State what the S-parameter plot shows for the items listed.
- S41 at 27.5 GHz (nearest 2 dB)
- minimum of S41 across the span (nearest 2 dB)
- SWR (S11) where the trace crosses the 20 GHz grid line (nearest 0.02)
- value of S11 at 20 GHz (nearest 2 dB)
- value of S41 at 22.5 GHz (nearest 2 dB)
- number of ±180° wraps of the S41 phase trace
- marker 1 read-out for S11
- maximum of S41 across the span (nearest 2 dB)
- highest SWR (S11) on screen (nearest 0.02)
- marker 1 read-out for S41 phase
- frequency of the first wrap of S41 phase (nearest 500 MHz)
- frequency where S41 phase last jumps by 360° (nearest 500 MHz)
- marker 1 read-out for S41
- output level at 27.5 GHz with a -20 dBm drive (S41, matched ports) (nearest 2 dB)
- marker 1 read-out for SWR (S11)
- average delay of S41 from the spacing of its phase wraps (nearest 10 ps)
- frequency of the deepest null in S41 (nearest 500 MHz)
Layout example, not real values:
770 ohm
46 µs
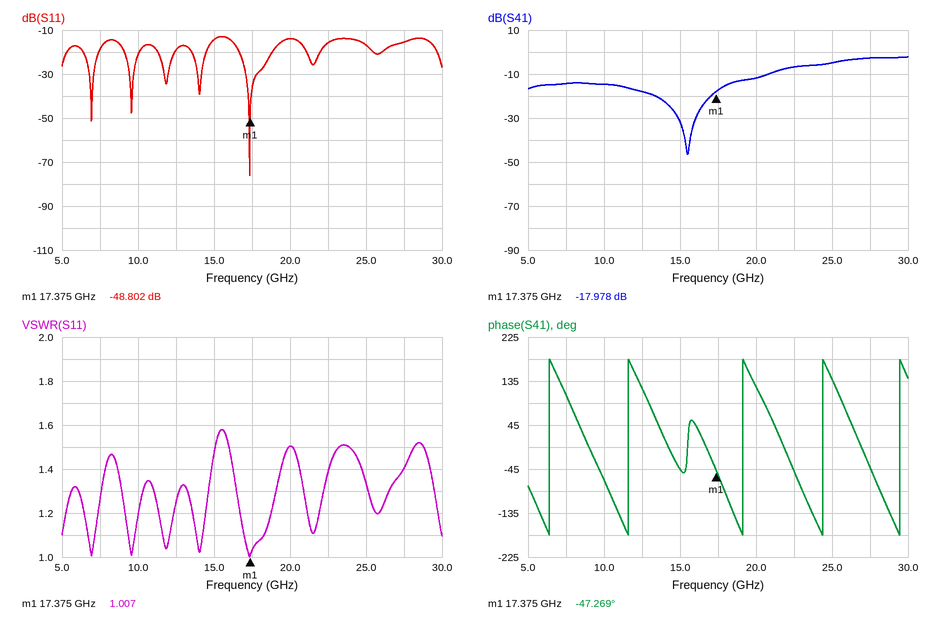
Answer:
-2 dB
-46 dB
1.50
-14 dB
-6 dB
5
-48.802 dB
-2 dB
1.58
-47.269°
6.5 GHz
29.5 GHz
-17.978 dB
-22 dBm
1.007
170 ps
15.5 GHz
